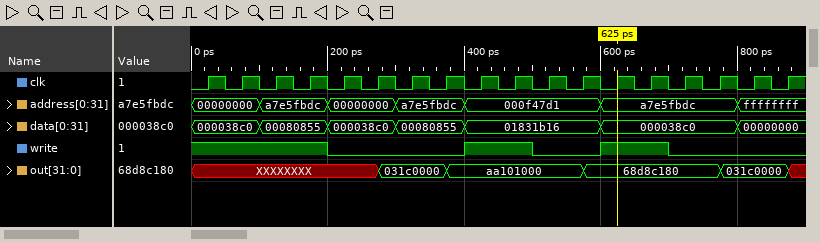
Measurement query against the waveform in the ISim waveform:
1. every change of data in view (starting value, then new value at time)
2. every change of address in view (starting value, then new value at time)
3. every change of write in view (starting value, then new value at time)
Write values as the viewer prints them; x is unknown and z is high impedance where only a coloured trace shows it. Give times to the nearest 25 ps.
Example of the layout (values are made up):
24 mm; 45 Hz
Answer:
000038c0, 00080855 at 100 ps, 000038c0 at 200 ps, 00080855 at 300 ps, 01831b16 at 400 ps, 000038c0 at 600 ps, 00000000 at 800 ps; 00000000, a7e5fbdc at 100 ps, 00000000 at 200 ps, a7e5fbdc at 300 ps, 000f47d1 at 400 ps, a7e5fbdc at 600 ps, ffffffff at 800 ps; 1, 0 at 200 ps, 1 at 400 ps, 0 at 500 ps, 1 at 600 ps, 0 at 700 ps
